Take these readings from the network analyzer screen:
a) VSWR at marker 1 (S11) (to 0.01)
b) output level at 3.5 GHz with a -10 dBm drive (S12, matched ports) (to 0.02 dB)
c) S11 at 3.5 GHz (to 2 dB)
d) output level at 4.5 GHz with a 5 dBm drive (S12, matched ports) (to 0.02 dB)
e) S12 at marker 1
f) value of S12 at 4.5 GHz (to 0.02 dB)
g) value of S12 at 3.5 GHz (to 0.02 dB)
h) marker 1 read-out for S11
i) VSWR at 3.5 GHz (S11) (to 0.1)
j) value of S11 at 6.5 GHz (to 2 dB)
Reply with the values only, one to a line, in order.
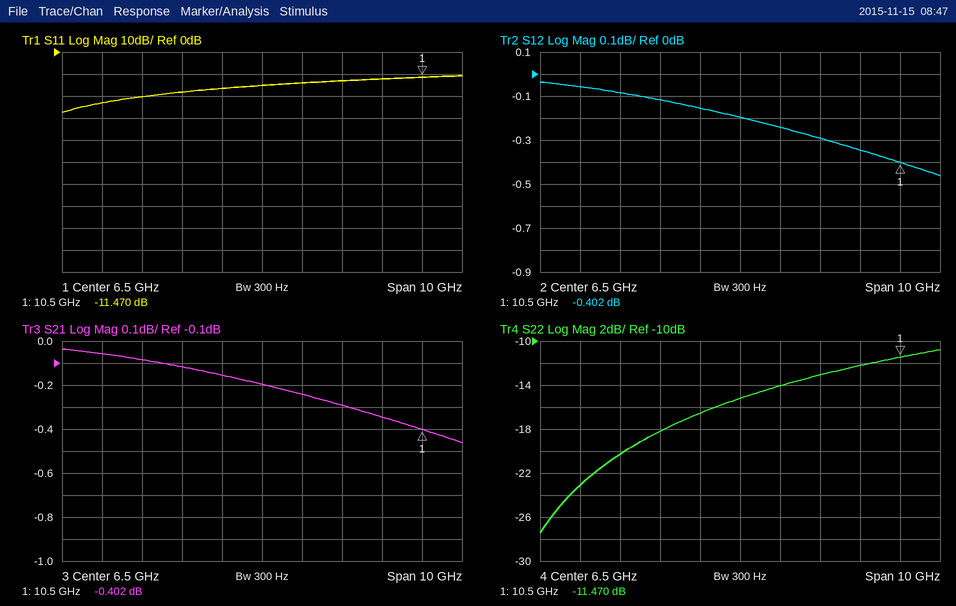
1.73
-10.08 dBm
-20 dB
4.88 dBm
-0.402 dB
-0.12 dB
-0.08 dB
-11.470 dB
1.2
-16 dB
